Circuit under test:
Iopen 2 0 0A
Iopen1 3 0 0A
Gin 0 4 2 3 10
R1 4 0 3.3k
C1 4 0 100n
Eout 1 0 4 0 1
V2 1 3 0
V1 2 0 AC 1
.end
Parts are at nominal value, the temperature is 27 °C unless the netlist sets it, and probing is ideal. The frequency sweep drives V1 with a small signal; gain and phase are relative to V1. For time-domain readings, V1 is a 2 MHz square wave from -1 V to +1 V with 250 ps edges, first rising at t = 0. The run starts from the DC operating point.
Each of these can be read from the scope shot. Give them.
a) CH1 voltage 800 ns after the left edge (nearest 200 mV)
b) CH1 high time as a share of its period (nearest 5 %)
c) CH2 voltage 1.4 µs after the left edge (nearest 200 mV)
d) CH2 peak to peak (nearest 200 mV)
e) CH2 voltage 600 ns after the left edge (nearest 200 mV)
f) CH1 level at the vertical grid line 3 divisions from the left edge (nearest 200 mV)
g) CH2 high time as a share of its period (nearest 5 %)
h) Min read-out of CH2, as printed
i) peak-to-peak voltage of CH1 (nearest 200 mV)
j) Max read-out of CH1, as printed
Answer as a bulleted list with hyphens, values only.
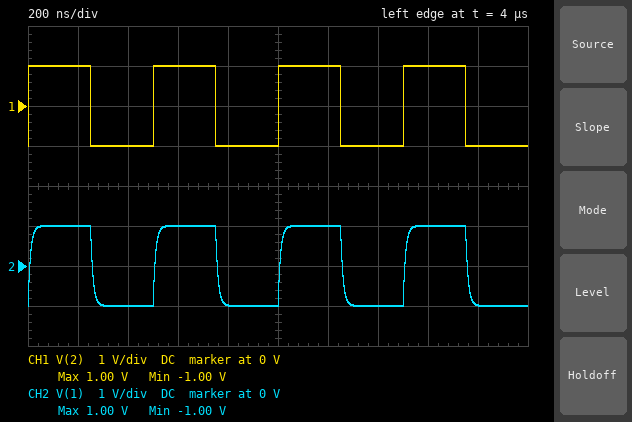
- -1.0 V
- 50 %
- -1.0 V
- 2.0 V
- 1.0 V
- 1.0 V
- 50 %
- -1.00 V
- 2.0 V
- 1.00 V
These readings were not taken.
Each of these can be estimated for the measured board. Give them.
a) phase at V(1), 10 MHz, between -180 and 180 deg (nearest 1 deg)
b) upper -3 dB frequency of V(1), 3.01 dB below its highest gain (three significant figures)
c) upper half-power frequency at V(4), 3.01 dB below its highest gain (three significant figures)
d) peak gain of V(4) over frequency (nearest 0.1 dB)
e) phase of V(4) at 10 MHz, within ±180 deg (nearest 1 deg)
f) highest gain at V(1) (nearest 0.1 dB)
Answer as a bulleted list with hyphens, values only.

- -32 deg
- 15.9 MHz
- 15.9 MHz
- 0 dB
- -32 deg
- 0 dB
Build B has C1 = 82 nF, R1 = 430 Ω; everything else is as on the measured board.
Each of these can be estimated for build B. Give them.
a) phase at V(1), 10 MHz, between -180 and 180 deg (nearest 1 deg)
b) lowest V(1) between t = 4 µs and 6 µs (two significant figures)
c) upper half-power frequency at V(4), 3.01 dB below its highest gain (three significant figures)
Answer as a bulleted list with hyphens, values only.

- -27 deg
- -1.0 V
- 19.4 MHz
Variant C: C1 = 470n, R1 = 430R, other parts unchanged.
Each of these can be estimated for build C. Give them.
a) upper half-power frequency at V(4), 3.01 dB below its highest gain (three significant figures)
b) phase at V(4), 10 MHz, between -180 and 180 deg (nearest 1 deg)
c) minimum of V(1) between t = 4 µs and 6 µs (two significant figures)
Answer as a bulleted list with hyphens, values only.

- 3.39 MHz
- -71 deg
- -990 mV
